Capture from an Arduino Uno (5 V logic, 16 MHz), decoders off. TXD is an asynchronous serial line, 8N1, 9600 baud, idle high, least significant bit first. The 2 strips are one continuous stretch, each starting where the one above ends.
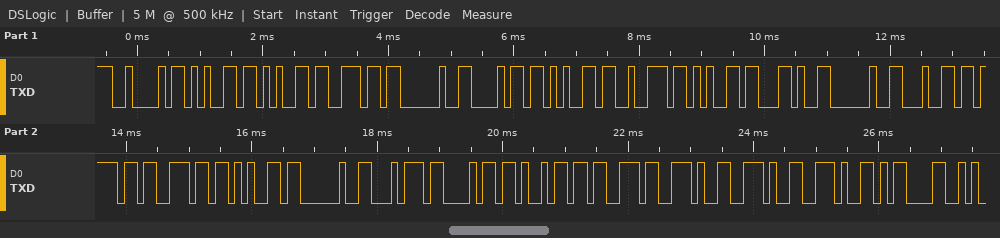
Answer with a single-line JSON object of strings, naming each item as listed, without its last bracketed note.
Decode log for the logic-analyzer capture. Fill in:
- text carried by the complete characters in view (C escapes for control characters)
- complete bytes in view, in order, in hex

{"text carried by the complete characters in view": "\"Been here, done this...\\r\"", "complete bytes in view, in order, in hex": "42 65 65 6E 20 68 65 72 65 2C 20 64 6F 6E 65 20 74 68 69 73 2E 2E 2E 0D"}
